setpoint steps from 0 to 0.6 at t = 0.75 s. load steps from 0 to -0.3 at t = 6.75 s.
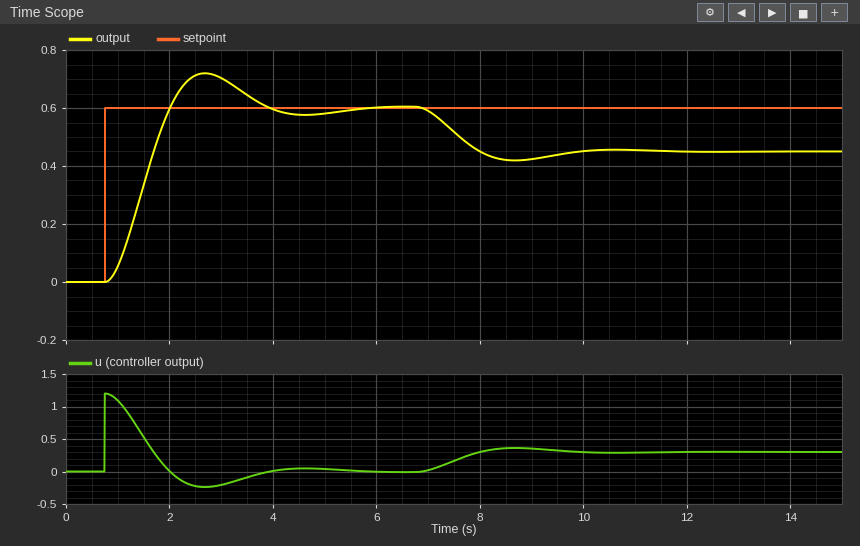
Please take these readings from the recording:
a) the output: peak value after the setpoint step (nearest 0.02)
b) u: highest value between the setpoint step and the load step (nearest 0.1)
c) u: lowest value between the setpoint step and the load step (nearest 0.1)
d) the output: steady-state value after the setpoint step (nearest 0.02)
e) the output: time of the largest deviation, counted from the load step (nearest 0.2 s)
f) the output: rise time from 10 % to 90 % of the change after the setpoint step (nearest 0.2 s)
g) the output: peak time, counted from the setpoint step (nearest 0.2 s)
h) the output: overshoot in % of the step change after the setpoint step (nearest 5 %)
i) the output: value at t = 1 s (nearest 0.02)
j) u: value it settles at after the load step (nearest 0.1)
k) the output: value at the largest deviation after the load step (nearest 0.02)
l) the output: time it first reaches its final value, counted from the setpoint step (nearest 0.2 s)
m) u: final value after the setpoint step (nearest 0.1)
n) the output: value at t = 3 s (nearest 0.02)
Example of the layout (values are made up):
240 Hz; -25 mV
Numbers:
0.72; 1.2; -0.2; 0.60; 2.0 s; 0.8 s; 2.0 s; 20 %; 0.06; 0.3; 0.42; 1.2 s; 0.0; 0.70
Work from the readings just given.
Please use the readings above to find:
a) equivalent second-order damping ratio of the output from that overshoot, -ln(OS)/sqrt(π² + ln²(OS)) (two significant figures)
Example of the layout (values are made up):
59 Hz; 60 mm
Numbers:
0.46
